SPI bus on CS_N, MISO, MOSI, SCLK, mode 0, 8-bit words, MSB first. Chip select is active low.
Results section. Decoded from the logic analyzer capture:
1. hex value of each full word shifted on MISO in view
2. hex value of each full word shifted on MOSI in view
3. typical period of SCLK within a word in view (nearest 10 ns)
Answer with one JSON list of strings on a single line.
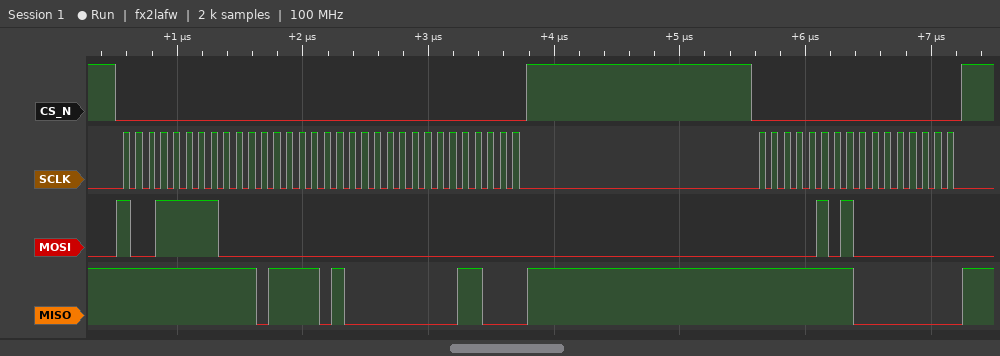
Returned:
["FF, EF, 40, 18, FF, 00", "9F, 00, 00, 00, 05, 00", "100 ns"]
